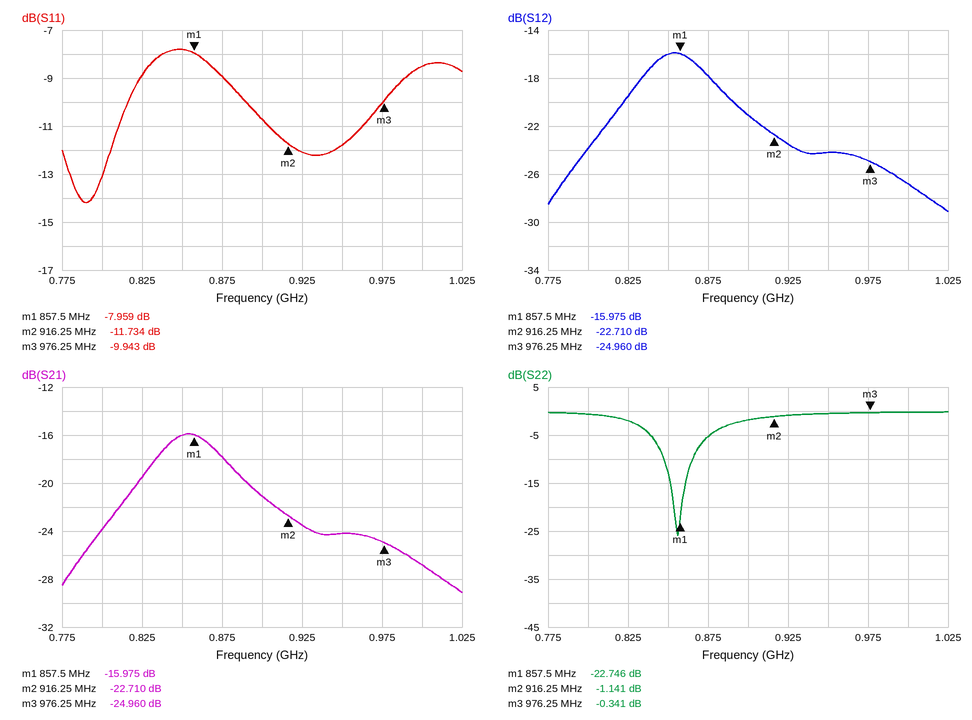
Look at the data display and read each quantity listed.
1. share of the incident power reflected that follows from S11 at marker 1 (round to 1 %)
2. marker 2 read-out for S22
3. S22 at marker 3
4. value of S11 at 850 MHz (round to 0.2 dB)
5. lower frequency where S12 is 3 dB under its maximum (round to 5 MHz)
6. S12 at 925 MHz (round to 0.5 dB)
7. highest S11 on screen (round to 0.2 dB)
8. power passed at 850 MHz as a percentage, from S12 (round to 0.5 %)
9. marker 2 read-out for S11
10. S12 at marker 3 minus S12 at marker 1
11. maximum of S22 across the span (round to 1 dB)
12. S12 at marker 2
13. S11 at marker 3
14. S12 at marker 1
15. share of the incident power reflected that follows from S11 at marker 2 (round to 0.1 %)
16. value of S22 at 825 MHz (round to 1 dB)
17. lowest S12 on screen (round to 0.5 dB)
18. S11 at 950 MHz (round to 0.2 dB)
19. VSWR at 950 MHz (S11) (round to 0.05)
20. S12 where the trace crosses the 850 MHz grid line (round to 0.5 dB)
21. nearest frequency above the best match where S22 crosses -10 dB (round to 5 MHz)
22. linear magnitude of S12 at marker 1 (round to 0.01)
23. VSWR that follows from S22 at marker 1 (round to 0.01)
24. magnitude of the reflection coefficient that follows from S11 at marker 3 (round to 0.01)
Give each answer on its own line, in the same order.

16 %
-1.141 dB
-0.341 dB
-7.8 dB
830 MHz
-23.5 dB
-7.8 dB
2.5 %
-11.734 dB
-8.985 dB
0 dB
-22.710 dB
-9.943 dB
-15.975 dB
6.7 %
-2 dB
-29.0 dB
-11.8 dB
1.70
-16.0 dB
865 MHz
0.16
1.16
0.32
